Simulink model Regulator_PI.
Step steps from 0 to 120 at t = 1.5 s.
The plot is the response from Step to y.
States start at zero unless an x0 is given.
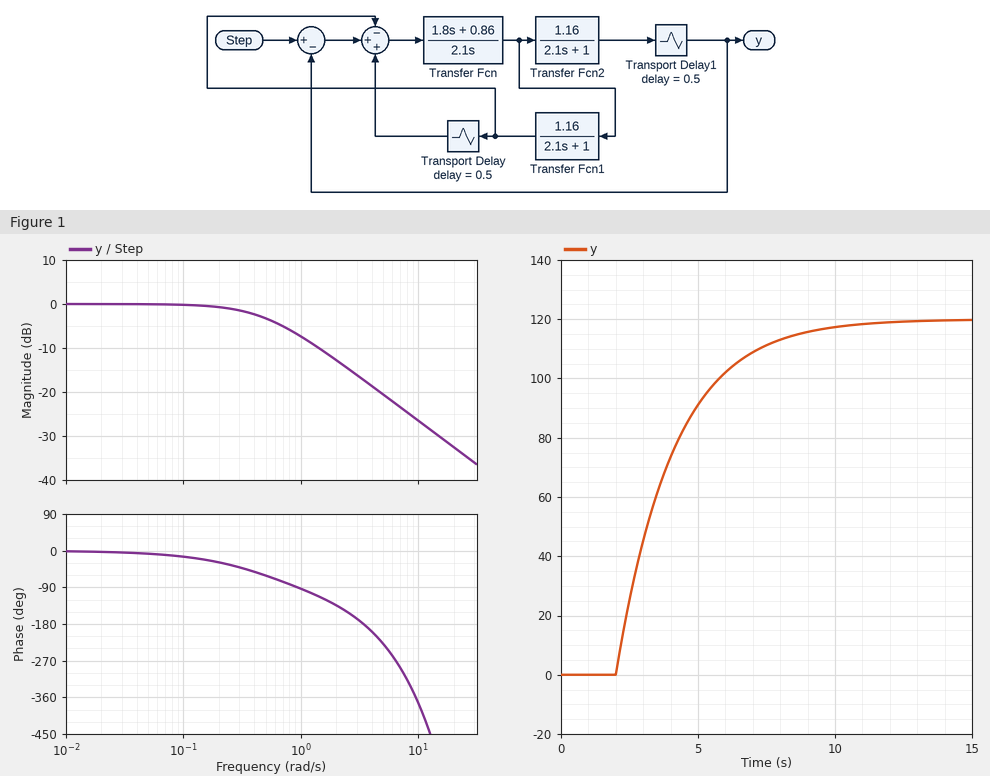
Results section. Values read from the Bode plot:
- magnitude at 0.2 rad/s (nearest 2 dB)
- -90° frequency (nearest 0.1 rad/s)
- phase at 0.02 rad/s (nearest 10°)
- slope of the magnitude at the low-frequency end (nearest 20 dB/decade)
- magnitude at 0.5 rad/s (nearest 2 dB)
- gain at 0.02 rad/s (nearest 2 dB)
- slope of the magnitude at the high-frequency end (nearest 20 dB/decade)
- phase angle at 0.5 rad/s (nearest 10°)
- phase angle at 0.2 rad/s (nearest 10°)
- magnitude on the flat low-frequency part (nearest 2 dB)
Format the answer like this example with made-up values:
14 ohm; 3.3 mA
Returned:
0 dB; 0.9 rad/s; 0°; 0 dB/decade; -4 dB; 0 dB; -20 dB/decade; -60°; -30°; 0 dB
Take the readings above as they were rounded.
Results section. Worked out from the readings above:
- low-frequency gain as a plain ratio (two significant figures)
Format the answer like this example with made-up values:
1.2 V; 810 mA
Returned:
1.0
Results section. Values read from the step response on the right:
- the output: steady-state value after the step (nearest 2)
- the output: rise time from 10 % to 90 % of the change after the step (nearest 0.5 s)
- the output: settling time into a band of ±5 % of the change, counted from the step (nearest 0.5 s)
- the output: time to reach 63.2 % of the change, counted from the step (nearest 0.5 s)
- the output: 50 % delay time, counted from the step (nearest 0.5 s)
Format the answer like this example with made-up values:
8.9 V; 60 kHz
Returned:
120; 4.5 s; 7.0 s; 2.5 s; 2.0 s
